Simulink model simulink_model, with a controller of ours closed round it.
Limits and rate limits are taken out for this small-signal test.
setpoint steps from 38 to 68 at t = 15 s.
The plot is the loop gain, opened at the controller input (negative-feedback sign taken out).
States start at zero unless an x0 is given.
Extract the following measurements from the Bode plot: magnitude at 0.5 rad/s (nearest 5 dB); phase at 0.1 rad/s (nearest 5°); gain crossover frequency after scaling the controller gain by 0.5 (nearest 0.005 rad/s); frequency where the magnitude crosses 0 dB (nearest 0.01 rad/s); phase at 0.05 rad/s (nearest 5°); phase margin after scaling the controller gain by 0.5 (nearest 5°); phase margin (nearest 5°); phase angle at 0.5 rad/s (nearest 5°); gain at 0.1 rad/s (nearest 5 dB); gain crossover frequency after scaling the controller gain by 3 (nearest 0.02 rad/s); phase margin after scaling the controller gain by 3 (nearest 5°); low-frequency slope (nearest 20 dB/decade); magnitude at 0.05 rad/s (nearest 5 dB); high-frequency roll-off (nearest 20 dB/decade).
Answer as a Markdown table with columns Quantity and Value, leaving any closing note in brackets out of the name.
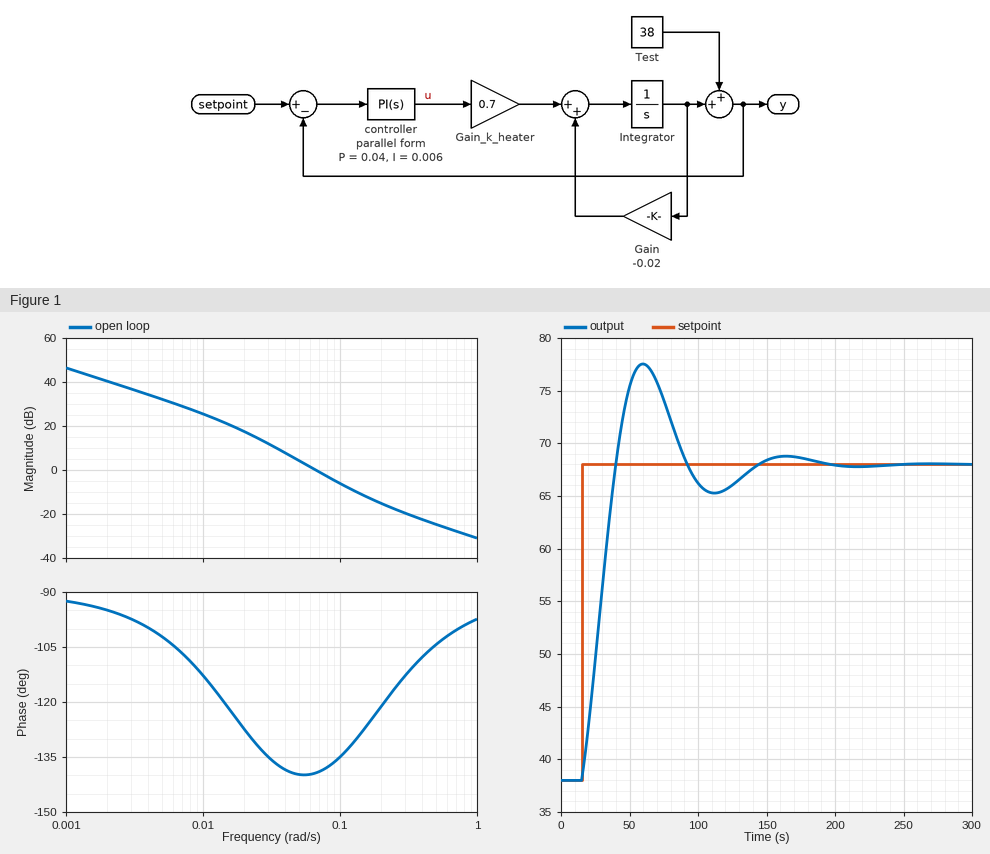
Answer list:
| Quantity | Value |
|---|---|
| magnitude at 0.5 rad/s | -25 dB |
| phase at 0.1 rad/s | -135° |
| gain crossover frequency after scaling the controller gain by 0.5 | 0.045 rad/s |
| frequency where the magnitude crosses 0 dB | 0.07 rad/s |
| phase at 0.05 rad/s | -140° |
| phase margin after scaling the controller gain by 0.5 | 40° |
| phase margin | 40° |
| phase angle at 0.5 rad/s | -105° |
| gain at 0.1 rad/s | -5 dB |
| gain crossover frequency after scaling the controller gain by 3 | 0.12 rad/s |
| phase margin after scaling the controller gain by 3 | 50° |
| low-frequency slope | -20 dB/decade |
| magnitude at 0.05 rad/s | 5 dB |
| high-frequency roll-off | -20 dB/decade |
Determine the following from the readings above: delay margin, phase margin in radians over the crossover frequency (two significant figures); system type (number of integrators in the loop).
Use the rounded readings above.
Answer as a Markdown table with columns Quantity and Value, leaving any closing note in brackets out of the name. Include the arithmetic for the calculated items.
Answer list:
| Quantity | Value |
|---|---|
| delay margin, phase margin in radians over the crossover frequency | 40 × π / 180 / 0.07 = 10.0 s |
| system type | 1 |
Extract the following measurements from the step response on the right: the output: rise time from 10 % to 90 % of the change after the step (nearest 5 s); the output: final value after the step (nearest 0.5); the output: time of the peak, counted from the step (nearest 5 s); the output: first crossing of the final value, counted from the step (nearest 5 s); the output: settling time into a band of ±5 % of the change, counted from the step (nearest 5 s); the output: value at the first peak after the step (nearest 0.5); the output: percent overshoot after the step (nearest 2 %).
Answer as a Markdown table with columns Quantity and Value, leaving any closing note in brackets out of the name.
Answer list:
| Quantity | Value |
|---|---|
| the output: rise time from 10 % to 90 % of the change after the step | 20 s |
| the output: final value after the step | 68.0 |
| the output: time of the peak, counted from the step | 45 s |
| the output: first crossing of the final value, counted from the step | 25 s |
| the output: settling time into a band of ±5 % of the change, counted from the step | 115 s |
| the output: value at the first peak after the step | 77.5 |
| the output: percent overshoot after the step | 32 % |
